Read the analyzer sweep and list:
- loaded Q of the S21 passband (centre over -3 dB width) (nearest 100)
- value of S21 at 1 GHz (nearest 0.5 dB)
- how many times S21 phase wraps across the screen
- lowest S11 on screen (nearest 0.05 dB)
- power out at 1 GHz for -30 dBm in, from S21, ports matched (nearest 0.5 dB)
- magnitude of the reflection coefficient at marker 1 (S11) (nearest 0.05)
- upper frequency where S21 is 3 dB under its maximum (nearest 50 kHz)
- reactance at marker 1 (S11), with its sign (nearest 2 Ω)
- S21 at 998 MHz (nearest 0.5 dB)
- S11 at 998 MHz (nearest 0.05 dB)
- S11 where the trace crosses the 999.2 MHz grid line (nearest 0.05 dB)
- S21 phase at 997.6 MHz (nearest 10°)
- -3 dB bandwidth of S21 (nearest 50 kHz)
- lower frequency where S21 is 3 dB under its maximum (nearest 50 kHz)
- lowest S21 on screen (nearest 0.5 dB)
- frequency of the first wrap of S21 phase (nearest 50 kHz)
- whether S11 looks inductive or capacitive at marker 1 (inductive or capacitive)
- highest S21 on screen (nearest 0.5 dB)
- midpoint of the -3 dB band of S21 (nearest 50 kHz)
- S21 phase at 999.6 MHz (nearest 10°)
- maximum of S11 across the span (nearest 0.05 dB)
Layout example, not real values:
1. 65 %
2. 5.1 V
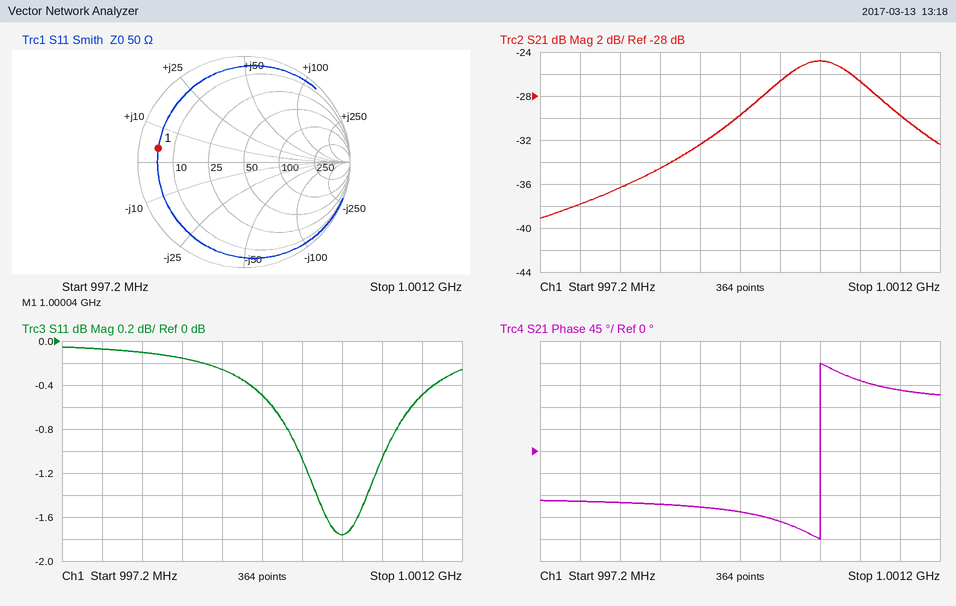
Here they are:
1. 900
2. -25.0 dB
3. 1
4. -1.75 dB
5. -55.0 dBm
6. 0.80
7. 1.00055 GHz
8. +4 Ω
9. -36.5 dB
10. -0.10 dB
11. -0.50 dB
12. -100°
13. 1.10 MHz
14. 999.45 MHz
15. -39.0 dB
16. 1.00000 GHz
17. inductive
18. -25.0 dB
19. 1.00000 GHz
20. -140°
21. -0.05 dB
